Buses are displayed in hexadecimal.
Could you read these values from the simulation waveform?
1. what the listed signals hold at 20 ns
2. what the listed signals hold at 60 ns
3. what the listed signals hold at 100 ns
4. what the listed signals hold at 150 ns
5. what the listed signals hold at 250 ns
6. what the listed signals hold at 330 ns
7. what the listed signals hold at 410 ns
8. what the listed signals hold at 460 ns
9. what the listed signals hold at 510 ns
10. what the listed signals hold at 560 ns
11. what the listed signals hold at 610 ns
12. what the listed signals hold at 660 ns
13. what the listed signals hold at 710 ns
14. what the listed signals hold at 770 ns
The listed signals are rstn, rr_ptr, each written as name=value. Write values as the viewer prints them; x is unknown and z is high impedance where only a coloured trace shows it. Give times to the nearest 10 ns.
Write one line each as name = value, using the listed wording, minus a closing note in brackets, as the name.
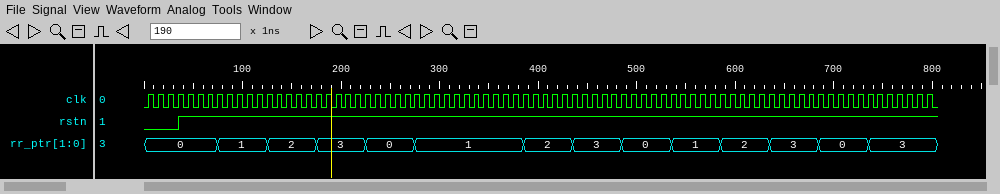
what the listed signals hold at 20 ns = rstn=0, rr_ptr=0
what the listed signals hold at 60 ns = rstn=1, rr_ptr=0
what the listed signals hold at 100 ns = rstn=1, rr_ptr=1
what the listed signals hold at 150 ns = rstn=1, rr_ptr=2
what the listed signals hold at 250 ns = rstn=1, rr_ptr=0
what the listed signals hold at 330 ns = rstn=1, rr_ptr=1
what the listed signals hold at 410 ns = rstn=1, rr_ptr=2
what the listed signals hold at 460 ns = rstn=1, rr_ptr=3
what the listed signals hold at 510 ns = rstn=1, rr_ptr=0
what the listed signals hold at 560 ns = rstn=1, rr_ptr=1
what the listed signals hold at 610 ns = rstn=1, rr_ptr=2
what the listed signals hold at 660 ns = rstn=1, rr_ptr=3
what the listed signals hold at 710 ns = rstn=1, rr_ptr=0
what the listed signals hold at 770 ns = rstn=1, rr_ptr=3
